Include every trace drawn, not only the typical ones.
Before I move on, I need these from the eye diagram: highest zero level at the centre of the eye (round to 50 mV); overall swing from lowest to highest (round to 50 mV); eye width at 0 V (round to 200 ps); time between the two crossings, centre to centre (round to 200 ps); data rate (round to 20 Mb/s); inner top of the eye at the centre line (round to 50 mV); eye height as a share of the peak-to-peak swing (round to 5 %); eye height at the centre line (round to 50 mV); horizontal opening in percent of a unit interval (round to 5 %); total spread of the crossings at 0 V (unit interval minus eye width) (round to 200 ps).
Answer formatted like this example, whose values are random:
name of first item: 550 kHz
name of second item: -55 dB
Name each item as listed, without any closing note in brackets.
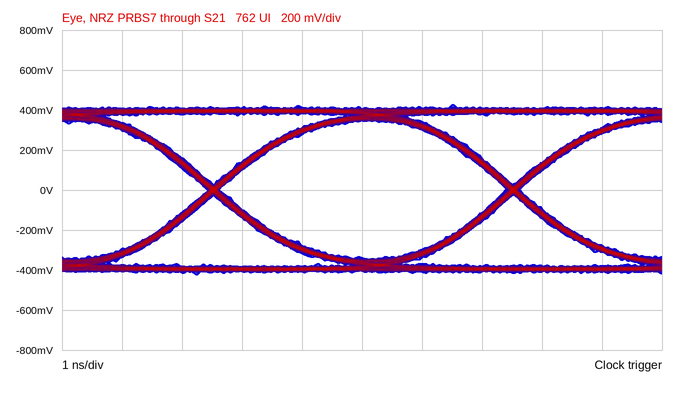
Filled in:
highest zero level at the centre of the eye: -350 mV
overall swing from lowest to highest: 850 mV
eye width at 0 V: 4.8 ns
time between the two crossings, centre to centre: 5.0 ns
data rate: 200 Mb/s
inner top of the eye at the centre line: 350 mV
eye height as a share of the peak-to-peak swing: 80 %
eye height at the centre line: 700 mV
horizontal opening in percent of a unit interval: 95 %
total spread of the crossings at 0 V (unit interval minus eye width): 200 ps
